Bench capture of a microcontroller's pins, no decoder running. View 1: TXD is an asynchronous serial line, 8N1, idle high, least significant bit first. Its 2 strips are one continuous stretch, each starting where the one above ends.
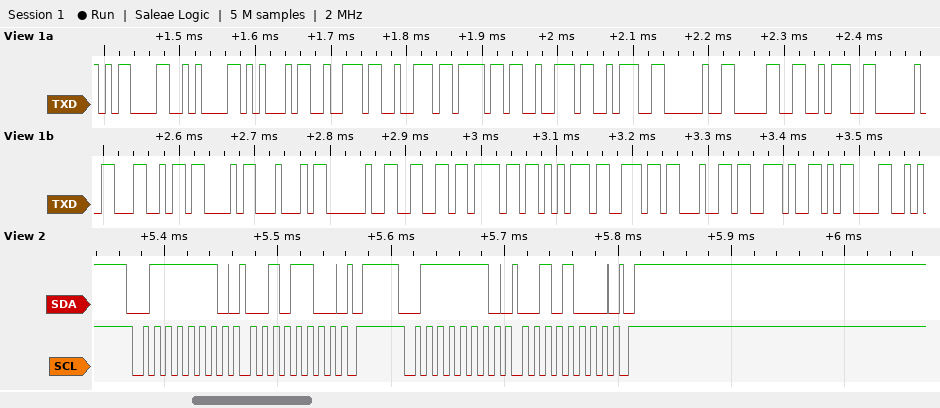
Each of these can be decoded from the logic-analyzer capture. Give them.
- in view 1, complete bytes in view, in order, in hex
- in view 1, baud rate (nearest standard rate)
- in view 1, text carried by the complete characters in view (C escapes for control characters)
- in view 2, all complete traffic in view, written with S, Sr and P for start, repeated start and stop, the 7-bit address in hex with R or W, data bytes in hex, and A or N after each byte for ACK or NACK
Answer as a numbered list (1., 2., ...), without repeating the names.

1. 0D 0A 45 72 72 6F 72 3A 20 30 3A 20 4C 43 44 20 66 6F 75 6E 64 2E 0D
2. 115200 baud
3. "\r\nError: 0: LCD found.\r"
4. S 3FW A 2C A P S 3FW A 28 A P
